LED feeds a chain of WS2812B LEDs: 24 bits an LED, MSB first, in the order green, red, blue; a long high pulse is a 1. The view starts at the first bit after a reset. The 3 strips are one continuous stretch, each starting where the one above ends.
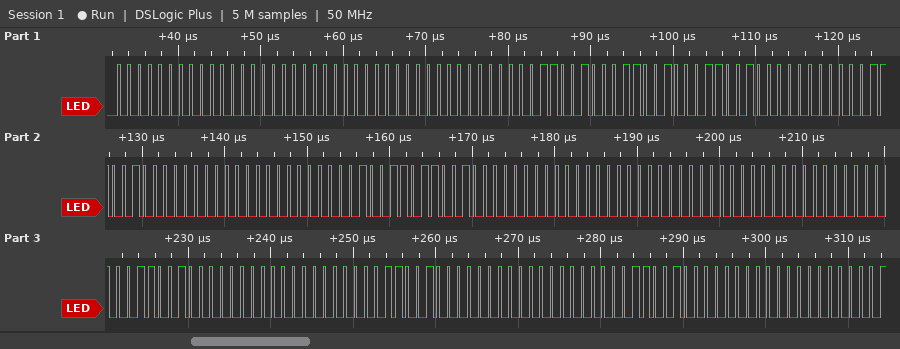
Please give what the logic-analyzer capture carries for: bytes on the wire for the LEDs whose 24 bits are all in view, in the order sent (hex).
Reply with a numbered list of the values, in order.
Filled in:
1. 00 00 00 00 00 64 64 64 00 64 00 00 13 64 00 00 00 00 00 64 00 00 64 00 00 64 00
